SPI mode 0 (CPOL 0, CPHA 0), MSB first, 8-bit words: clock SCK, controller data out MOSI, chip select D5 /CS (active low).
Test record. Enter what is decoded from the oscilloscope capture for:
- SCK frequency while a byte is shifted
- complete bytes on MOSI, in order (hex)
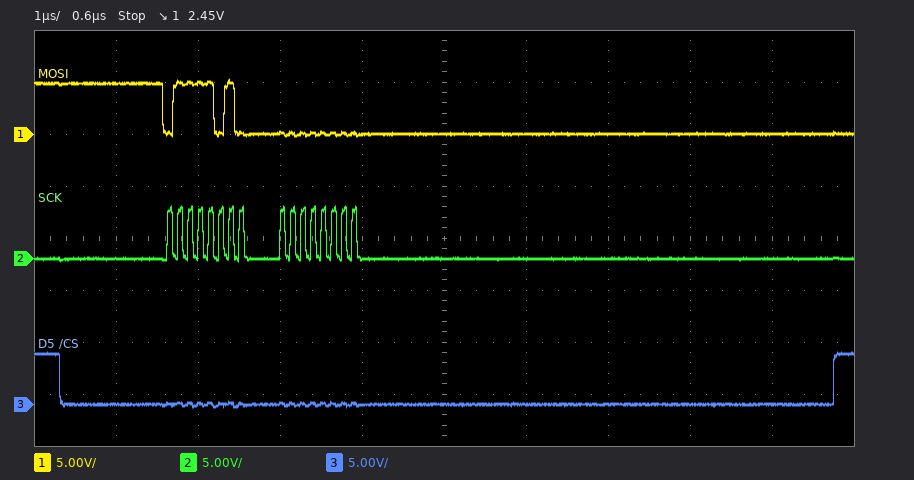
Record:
8 MHz
7A 00
